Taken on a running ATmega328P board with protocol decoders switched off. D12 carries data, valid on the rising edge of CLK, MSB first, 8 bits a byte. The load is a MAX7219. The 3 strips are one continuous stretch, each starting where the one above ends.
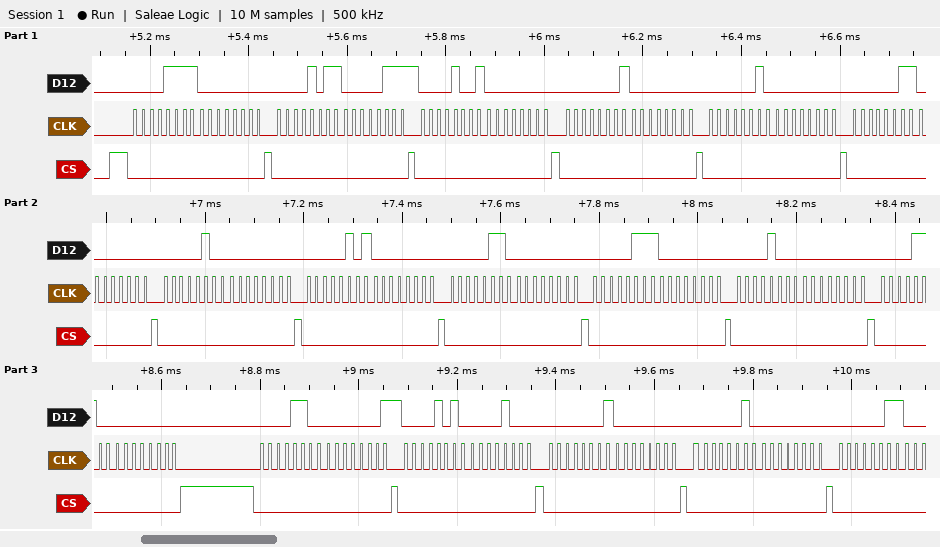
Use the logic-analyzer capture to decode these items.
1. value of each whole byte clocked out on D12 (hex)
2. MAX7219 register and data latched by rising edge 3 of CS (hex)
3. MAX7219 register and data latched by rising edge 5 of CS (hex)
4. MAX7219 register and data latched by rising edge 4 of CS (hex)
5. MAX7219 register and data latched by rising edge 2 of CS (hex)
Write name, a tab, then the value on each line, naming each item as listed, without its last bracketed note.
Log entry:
value of each whole byte clocked out on D12	0F 00 0B 07 09 00 01 00 02 00 03 00 04 00 05 00 06 00 07 00 08 00 0C 00 0C 01 0A 08 01 00 02 00 03
MAX7219 register and data latched by rising edge 3 of CS	register 0xB, data 0x07
MAX7219 register and data latched by rising edge 5 of CS	register 0x1, data 0x00
MAX7219 register and data latched by rising edge 4 of CS	register 0x9, data 0x00
MAX7219 register and data latched by rising edge 2 of CS	register 0xF, data 0x00
